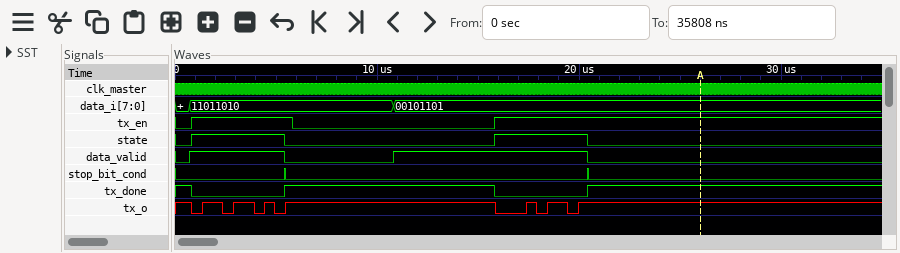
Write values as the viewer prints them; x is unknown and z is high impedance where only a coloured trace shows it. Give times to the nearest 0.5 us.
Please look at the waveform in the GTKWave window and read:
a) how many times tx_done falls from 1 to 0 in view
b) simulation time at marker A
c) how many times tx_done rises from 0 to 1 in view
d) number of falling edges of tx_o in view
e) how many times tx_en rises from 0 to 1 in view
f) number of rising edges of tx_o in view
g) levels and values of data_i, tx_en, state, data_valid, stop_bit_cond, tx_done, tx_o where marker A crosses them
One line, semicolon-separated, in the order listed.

2; 26 us; 2; 7; 2; 7; data_i=00101101, tx_en=1, state=0, data_valid=0, stop_bit_cond=0, tx_done=1, tx_o=1
